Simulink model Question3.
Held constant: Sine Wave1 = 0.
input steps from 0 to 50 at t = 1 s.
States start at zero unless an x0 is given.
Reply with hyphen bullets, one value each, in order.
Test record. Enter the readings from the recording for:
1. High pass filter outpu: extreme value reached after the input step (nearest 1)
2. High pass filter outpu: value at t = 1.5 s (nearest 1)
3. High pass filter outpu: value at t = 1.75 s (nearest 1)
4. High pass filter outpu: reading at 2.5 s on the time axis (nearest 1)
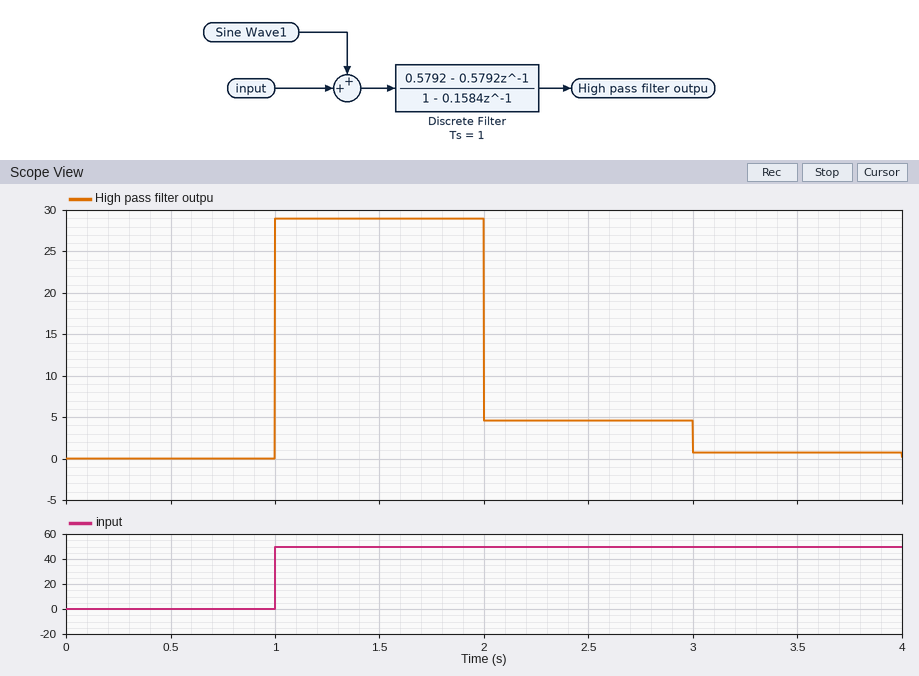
- 29
- 29
- 29
- 5
